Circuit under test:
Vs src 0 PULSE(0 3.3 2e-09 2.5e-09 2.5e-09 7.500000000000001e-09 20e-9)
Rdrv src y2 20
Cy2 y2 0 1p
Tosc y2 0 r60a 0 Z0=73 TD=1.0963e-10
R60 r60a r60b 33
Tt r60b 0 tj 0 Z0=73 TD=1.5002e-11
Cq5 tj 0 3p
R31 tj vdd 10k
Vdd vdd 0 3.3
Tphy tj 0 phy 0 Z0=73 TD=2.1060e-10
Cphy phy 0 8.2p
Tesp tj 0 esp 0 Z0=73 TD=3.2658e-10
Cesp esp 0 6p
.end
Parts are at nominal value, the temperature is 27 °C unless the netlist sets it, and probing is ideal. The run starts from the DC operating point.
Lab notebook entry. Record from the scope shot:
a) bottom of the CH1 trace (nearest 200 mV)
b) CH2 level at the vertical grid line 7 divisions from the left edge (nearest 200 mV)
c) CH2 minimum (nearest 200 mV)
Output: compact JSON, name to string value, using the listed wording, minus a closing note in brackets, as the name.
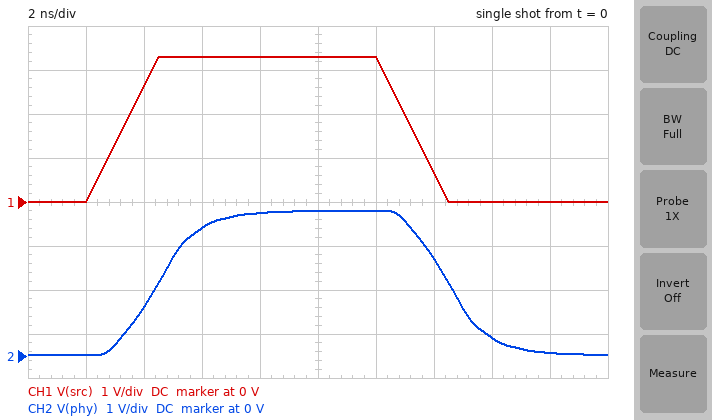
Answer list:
{"bottom of the CH1 trace": "0 V", "CH2 level at the vertical grid line 7 divisions from the left edge": "2.2 V", "CH2 minimum": "0 V"}
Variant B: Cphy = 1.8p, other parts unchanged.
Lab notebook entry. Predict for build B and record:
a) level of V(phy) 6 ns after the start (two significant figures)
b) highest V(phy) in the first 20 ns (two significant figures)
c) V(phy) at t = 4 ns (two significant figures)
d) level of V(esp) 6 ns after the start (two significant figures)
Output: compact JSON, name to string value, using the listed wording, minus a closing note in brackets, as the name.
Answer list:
{"level of V(phy) 6 ns after the start": "3.1 V", "highest V(phy) in the first 20 ns": "3.4 V", "V(phy) at t = 4 ns": "1.3 V", "level of V(esp) 6 ns after the start": "3.3 V"}
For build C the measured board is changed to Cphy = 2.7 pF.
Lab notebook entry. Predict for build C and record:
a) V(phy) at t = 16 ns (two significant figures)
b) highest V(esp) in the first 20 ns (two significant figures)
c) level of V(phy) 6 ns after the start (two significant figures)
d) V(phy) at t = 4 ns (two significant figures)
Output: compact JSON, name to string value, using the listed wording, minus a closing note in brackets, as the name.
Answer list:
{"V(phy) at t = 16 ns": "270 mV", "highest V(esp) in the first 20 ns": "3.4 V", "level of V(phy) 6 ns after the start": "3.0 V", "V(phy) at t = 4 ns": "1.3 V"}
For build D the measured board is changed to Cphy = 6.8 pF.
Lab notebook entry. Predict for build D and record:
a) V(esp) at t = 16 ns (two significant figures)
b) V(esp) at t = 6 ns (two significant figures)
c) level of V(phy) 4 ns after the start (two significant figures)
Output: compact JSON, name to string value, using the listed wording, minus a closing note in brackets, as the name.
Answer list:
{"V(esp) at t = 16 ns": "340 mV", "V(esp) at t = 6 ns": "3.0 V", "level of V(phy) 4 ns after the start": "1.2 V"}
